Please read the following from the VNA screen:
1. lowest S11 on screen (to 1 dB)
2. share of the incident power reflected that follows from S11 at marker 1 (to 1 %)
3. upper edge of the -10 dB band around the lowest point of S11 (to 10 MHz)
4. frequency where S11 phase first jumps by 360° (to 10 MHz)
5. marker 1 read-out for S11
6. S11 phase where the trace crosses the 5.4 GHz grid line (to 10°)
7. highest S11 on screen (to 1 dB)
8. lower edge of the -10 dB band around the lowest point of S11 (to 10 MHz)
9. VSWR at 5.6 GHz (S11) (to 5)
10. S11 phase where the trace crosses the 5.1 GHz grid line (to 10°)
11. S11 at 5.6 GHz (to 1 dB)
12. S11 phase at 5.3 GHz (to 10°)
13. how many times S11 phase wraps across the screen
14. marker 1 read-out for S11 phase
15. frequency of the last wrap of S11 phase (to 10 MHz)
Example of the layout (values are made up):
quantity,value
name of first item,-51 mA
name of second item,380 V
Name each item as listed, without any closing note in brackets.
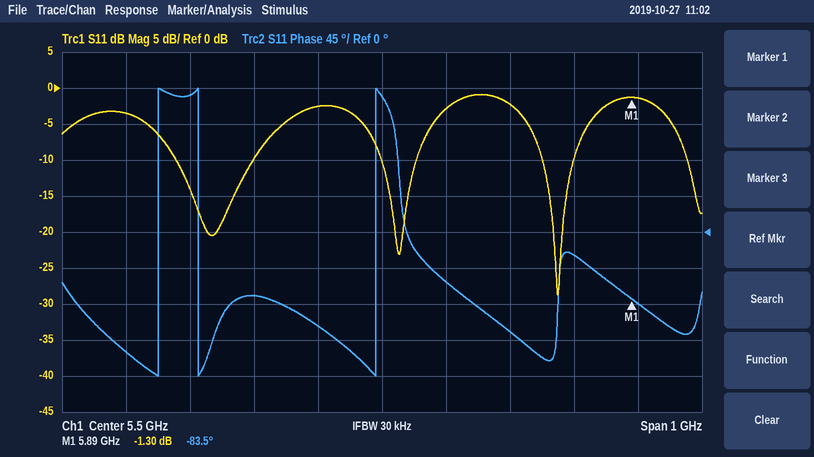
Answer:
quantity,value
lowest S11 on screen,-29 dB
share of the incident power reflected that follows from S11 at marker 1,74 %
upper edge of the -10 dB band around the lowest point of S11,5.80 GHz
frequency where S11 phase first jumps by 360°,5.15 GHz
marker 1 read-out for S11,-1.30 dB
S11 phase where the trace crosses the 5.4 GHz grid line,-120°
highest S11 on screen,-1 dB
lower edge of the -10 dB band around the lowest point of S11,5.75 GHz
VSWR at 5.6 GHz (S11),5
S11 phase where the trace crosses the 5.1 GHz grid line,-150°
S11 at 5.6 GHz,-3 dB
S11 phase at 5.3 GHz,-80°
how many times S11 phase wraps across the screen,3
marker 1 read-out for S11 phase,-83.5°
frequency of the last wrap of S11 phase,5.49 GHz
